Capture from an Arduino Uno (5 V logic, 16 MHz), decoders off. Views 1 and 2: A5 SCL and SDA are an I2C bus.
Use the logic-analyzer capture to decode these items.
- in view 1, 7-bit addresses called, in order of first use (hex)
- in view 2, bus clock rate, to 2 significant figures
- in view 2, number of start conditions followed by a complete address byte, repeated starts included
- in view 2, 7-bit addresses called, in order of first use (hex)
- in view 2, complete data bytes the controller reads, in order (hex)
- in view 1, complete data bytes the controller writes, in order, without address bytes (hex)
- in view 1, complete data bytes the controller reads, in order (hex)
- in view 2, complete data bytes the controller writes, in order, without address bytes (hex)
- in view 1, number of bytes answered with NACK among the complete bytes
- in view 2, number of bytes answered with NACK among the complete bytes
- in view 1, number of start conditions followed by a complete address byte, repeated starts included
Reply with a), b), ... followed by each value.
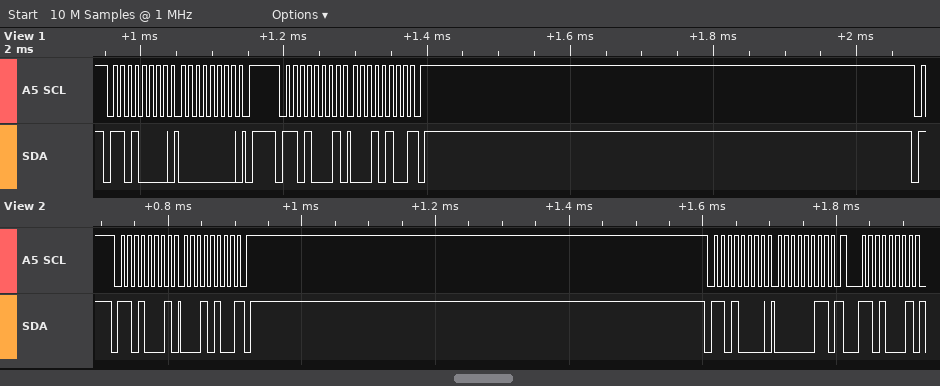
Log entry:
a) 0x68
b) 100 kHz
c) 3
d) 0x68
e) 14
f) 00
g) 14
h) 03
i) 1
j) 1
k) 2
